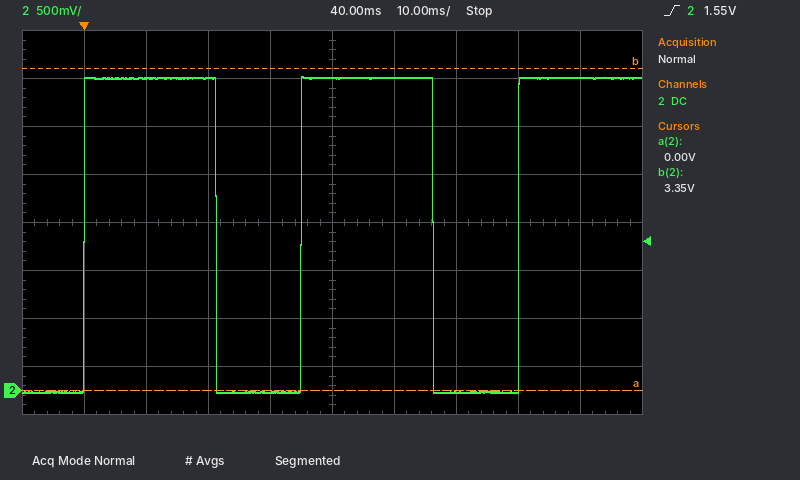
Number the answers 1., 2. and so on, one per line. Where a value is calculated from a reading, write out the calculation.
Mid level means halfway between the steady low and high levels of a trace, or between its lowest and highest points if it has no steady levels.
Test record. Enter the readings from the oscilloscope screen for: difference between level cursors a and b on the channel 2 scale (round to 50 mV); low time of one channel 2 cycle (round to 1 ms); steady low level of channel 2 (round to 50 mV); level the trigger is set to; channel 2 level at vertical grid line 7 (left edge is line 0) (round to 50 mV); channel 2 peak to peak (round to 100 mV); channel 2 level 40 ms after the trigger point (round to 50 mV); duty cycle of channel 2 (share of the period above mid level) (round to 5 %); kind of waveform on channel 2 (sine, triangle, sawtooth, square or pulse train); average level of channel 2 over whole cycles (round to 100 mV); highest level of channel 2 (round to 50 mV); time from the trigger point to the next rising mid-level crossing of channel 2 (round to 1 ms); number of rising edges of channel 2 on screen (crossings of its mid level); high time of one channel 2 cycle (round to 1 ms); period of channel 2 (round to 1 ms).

1. 3.35 V
2. 14 ms
3. 0 mV
4. 1.55 V
5. 0 mV
6. 3.30 V
7. 3.25 V
8. 21 ms / 35 ms ≈ 60 %
9. pulse train
10. 0 mV + 0.6 × (3.25 V − (0 mV)) ≈ 2.0 V
11. 3.25 V
12. 35 ms
13. 3
14. 21 ms
15. 35 ms
